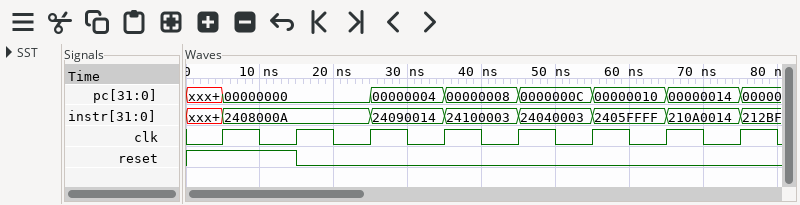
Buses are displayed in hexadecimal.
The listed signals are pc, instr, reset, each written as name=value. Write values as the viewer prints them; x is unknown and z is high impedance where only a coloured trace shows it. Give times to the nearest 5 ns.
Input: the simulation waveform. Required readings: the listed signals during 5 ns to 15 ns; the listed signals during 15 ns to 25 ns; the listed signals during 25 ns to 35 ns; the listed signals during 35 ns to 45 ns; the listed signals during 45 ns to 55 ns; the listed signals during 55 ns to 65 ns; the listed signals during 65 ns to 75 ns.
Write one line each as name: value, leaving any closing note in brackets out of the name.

the listed signals during 5 ns to 15 ns: pc=00000000, instr=2408000A, reset=1
the listed signals during 15 ns to 25 ns: pc=00000000, instr=2408000A, reset=0
the listed signals during 25 ns to 35 ns: pc=00000004, instr=24090014, reset=0
the listed signals during 35 ns to 45 ns: pc=00000008, instr=24100003, reset=0
the listed signals during 45 ns to 55 ns: pc=0000000C, instr=24040003, reset=0
the listed signals during 55 ns to 65 ns: pc=00000010, instr=2405FFFF, reset=0
the listed signals during 65 ns to 75 ns: pc=00000014, instr=210A0014, reset=0
